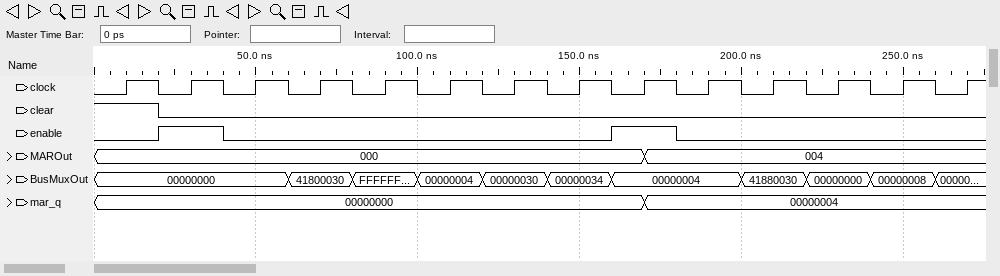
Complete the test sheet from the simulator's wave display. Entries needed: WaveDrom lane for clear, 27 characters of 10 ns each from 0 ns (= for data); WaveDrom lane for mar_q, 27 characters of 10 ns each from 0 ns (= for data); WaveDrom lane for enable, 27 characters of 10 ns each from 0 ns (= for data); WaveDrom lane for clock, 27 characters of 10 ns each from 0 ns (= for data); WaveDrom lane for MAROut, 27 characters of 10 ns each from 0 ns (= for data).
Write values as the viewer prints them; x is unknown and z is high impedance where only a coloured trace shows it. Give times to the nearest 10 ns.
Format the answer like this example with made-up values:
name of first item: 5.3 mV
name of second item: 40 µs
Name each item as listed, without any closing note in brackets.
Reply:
WaveDrom lane for clear, 27 characters of 10 ns each from 0 ns: {name: 'clear', wave: '1.0........................'}
WaveDrom lane for mar_q, 27 characters of 10 ns each from 0 ns: {name: 'mar_q', wave: '=................=.........', data: '00000000 00000004'}
WaveDrom lane for enable, 27 characters of 10 ns each from 0 ns: {name: 'enable', wave: '0.1.0...........1.0........'}
WaveDrom lane for clock, 27 characters of 10 ns each from 0 ns: {name: 'clock', wave: '010101010101010101010101010'}
WaveDrom lane for MAROut, 27 characters of 10 ns each from 0 ns: {name: 'MAROut', wave: '=................=.........', data: '000 004'}
